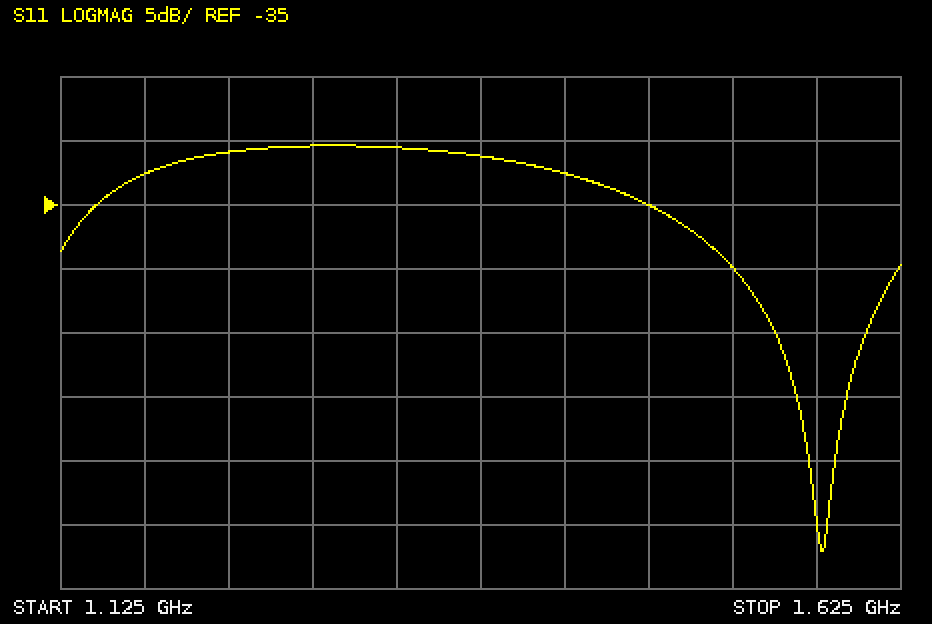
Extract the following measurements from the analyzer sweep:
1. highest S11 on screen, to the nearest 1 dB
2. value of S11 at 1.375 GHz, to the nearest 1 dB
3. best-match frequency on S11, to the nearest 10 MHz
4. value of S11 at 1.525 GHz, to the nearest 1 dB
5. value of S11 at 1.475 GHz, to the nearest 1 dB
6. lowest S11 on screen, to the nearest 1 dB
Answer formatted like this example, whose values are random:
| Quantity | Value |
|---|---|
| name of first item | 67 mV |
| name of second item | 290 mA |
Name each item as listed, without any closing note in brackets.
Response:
| Quantity | Value |
|---|---|
| highest S11 on screen, to the nearest 1 dB | -30 dB |
| value of S11 at 1.375 GHz, to the nearest 1 dB | -31 dB |
| best-match frequency on S11, to the nearest 10 MHz | 1.58 GHz |
| value of S11 at 1.525 GHz, to the nearest 1 dB | -40 dB |
| value of S11 at 1.475 GHz, to the nearest 1 dB | -35 dB |
| lowest S11 on screen, to the nearest 1 dB | -62 dB |
